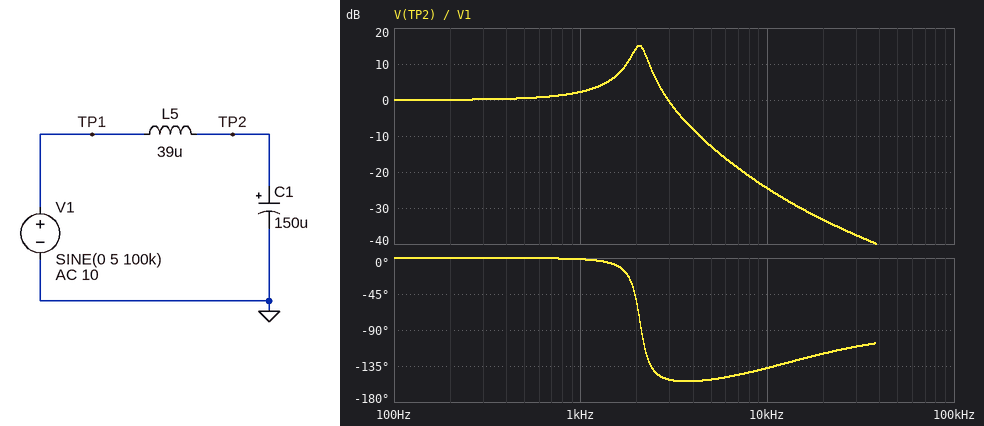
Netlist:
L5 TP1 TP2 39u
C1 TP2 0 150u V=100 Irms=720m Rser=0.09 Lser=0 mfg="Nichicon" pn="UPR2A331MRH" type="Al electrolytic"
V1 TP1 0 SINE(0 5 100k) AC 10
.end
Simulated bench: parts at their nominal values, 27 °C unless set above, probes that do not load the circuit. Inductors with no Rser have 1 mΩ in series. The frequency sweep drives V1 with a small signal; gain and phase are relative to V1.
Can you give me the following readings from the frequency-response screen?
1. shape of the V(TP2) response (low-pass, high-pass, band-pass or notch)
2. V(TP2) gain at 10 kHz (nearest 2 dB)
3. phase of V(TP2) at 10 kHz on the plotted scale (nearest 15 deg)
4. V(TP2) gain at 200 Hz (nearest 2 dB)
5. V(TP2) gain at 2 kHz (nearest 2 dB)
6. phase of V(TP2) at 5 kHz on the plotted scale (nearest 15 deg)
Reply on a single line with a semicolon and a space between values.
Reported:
low-pass; -24 dB; -135 deg; 0 dB; 14 dB; -150 deg
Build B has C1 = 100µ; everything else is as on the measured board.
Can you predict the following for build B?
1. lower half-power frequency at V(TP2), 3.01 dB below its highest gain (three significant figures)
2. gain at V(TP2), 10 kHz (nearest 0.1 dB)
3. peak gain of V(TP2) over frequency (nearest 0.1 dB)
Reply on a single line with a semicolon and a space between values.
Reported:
2.34 kHz; -22.0 dB; 16.8 dB
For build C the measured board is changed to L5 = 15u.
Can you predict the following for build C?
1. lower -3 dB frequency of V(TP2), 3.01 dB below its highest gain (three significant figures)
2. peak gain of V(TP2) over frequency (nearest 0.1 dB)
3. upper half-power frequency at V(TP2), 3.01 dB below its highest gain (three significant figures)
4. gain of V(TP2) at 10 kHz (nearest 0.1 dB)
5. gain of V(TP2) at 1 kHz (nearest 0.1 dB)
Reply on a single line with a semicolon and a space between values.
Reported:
2.77 kHz; 11.2 dB; 3.75 kHz; -15.6 dB; 0.8 dB
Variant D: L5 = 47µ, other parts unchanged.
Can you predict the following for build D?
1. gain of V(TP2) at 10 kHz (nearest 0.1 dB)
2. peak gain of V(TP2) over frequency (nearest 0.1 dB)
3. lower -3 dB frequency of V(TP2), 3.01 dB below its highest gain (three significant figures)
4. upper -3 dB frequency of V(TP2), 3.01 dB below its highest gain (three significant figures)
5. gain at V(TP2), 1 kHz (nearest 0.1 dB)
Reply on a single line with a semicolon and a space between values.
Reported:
-26.2 dB; 15.9 dB; 1.72 kHz; 2.03 kHz; 2.8 dB
